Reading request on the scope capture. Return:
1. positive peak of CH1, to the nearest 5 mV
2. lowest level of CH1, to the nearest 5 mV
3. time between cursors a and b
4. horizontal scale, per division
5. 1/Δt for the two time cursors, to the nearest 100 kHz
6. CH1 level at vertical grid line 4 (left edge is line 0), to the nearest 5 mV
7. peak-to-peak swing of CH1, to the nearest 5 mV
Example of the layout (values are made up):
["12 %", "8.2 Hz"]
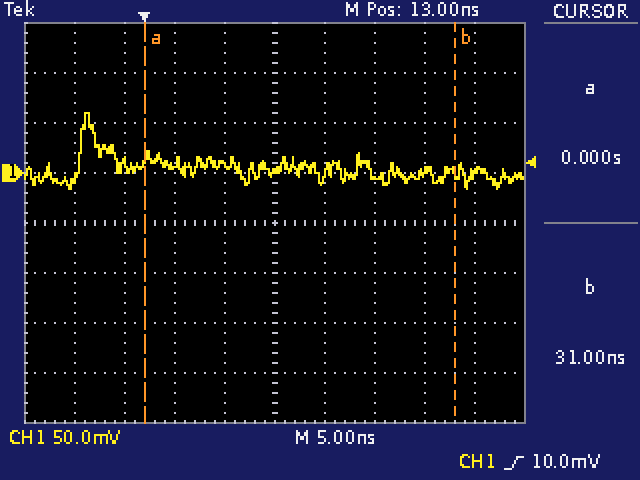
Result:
["60 mV", "-15 mV", "31.0 ns", "5 ns", "32.3 MHz", "10 mV", "75 mV"]
